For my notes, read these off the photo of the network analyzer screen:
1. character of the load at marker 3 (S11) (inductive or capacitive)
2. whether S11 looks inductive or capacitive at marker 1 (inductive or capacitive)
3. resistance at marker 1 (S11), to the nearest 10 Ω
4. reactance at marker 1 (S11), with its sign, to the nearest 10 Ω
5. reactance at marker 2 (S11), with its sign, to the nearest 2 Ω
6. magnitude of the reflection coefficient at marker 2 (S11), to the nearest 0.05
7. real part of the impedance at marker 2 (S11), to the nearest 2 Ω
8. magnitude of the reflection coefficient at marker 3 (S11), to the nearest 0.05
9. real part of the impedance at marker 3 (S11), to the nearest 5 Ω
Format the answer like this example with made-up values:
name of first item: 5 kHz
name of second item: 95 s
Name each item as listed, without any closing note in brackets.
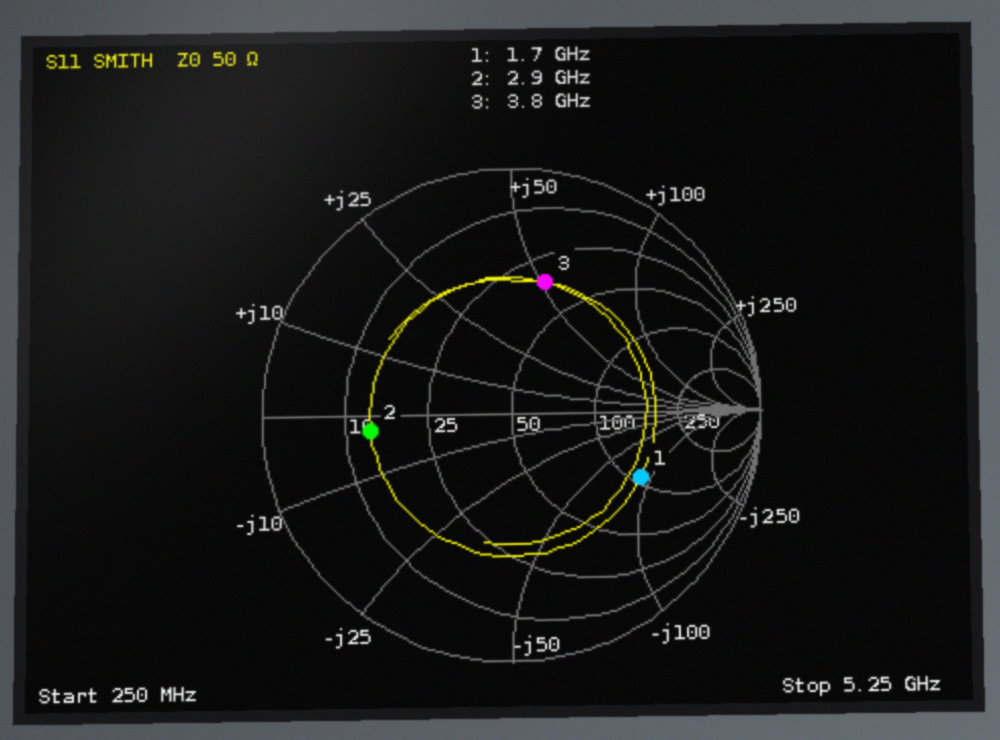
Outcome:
character of the load at marker 3 (S11): inductive
whether S11 looks inductive or capacitive at marker 1: capacitive
resistance at marker 1 (S11), to the nearest 10 Ω: 110 Ω
reactance at marker 1 (S11), with its sign, to the nearest 10 Ω: -90 Ω
reactance at marker 2 (S11), with its sign, to the nearest 2 Ω: -2 Ω
magnitude of the reflection coefficient at marker 2 (S11), to the nearest 0.05: 0.55
real part of the impedance at marker 2 (S11), to the nearest 2 Ω: 14 Ω
magnitude of the reflection coefficient at marker 3 (S11), to the nearest 0.05: 0.55
real part of the impedance at marker 3 (S11), to the nearest 5 Ω: 35 Ω
